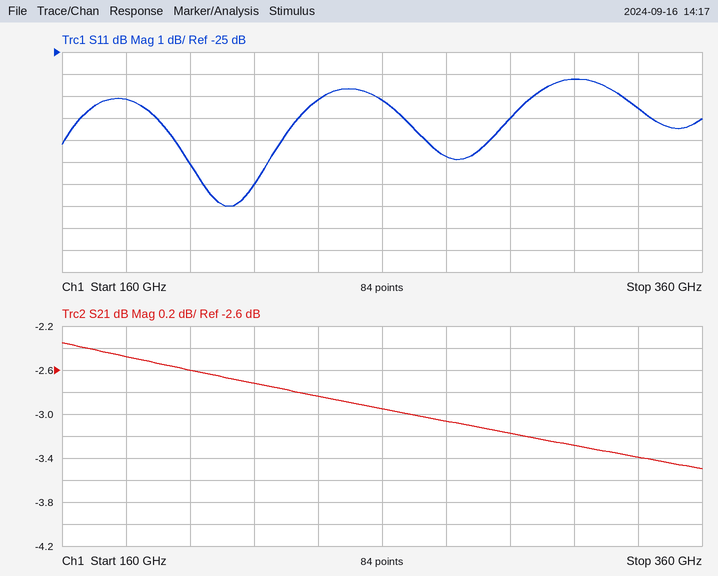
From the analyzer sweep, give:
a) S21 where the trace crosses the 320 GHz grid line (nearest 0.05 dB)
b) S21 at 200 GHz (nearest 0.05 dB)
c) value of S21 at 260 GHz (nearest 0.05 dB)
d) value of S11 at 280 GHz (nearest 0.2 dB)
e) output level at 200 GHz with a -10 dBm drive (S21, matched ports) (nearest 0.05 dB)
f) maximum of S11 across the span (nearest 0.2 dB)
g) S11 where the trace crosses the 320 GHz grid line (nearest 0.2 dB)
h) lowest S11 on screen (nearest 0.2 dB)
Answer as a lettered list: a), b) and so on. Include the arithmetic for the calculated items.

a) -3.30 dB
b) -2.60 dB
c) -2.95 dB
d) -29.8 dB
e) -10 dBm + (-2.60 dB) = -12.60 dBm
f) -26.2 dB
g) -26.2 dB
h) -32.0 dB
